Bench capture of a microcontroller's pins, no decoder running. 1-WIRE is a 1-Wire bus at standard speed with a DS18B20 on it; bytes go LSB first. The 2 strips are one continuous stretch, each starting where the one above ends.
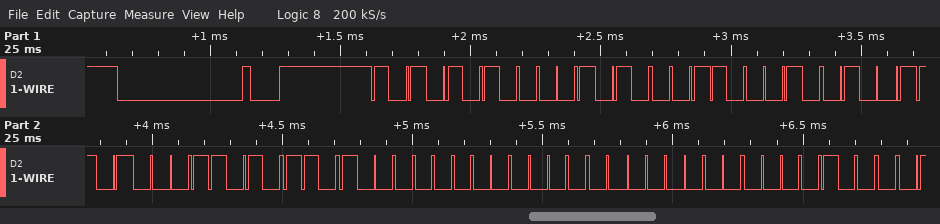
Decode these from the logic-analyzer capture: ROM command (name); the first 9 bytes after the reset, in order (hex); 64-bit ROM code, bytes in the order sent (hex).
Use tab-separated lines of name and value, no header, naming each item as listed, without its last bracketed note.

ROM command	Match ROM
the first 9 bytes after the reset, in order	55 28 46 B2 58 0B 00 00 10
64-bit ROM code, bytes in the order sent	28 46 B2 58 0B 00 00 10
